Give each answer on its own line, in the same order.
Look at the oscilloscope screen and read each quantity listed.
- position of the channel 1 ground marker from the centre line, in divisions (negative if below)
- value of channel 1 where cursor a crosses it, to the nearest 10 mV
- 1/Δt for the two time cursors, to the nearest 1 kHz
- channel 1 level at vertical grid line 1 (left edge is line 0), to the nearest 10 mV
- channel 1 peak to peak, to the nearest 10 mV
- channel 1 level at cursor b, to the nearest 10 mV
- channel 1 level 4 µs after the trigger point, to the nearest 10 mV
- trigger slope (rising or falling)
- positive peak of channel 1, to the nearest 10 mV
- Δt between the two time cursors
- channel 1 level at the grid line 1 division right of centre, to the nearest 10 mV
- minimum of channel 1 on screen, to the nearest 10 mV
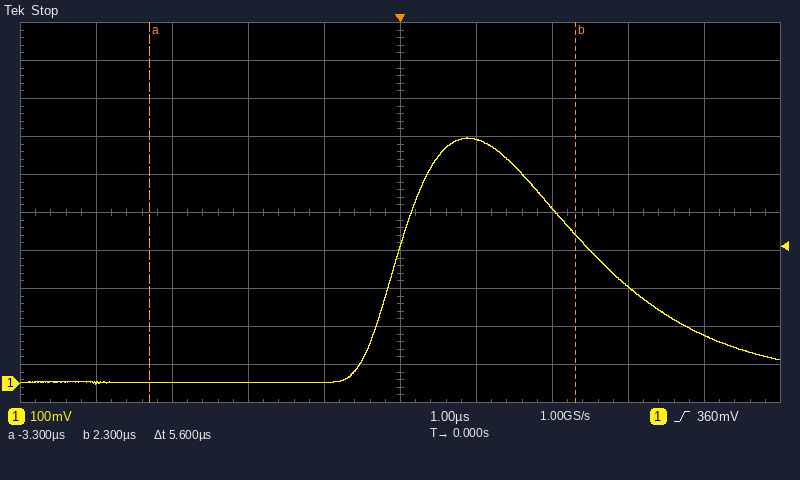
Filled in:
-4.5 div
0 mV
179 kHz
0 mV
650 mV
390 mV
130 mV
rising
650 mV
5.6 µs
640 mV
0 mV
